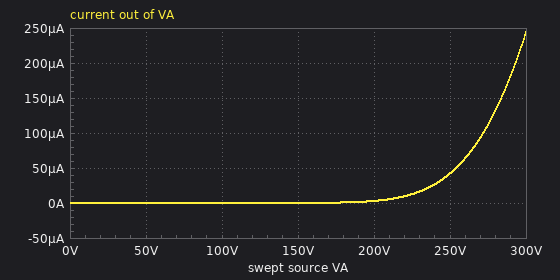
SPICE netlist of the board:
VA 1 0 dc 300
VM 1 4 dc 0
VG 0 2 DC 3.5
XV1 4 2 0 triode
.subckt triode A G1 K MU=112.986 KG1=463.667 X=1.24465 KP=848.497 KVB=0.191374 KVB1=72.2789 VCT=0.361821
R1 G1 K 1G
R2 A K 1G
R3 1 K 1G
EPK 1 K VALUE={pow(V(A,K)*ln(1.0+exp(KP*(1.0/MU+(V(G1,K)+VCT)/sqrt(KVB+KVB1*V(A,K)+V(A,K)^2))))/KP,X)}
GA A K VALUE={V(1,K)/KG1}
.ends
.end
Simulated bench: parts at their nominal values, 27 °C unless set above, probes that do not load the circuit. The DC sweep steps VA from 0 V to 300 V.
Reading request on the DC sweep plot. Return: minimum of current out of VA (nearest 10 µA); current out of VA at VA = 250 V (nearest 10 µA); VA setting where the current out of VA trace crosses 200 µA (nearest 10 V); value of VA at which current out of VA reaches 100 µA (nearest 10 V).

0 A
40 µA
290 V
270 V
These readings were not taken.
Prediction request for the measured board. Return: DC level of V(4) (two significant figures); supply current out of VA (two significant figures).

300 V
240 µA
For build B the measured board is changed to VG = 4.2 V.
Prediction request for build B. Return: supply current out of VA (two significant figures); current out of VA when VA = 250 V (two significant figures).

35 µA
3.6 µA
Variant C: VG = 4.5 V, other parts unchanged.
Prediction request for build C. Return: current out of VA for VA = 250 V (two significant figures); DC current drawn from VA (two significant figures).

1.4 µA
14 µA
